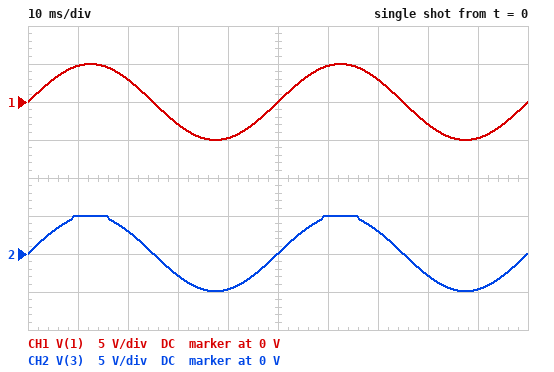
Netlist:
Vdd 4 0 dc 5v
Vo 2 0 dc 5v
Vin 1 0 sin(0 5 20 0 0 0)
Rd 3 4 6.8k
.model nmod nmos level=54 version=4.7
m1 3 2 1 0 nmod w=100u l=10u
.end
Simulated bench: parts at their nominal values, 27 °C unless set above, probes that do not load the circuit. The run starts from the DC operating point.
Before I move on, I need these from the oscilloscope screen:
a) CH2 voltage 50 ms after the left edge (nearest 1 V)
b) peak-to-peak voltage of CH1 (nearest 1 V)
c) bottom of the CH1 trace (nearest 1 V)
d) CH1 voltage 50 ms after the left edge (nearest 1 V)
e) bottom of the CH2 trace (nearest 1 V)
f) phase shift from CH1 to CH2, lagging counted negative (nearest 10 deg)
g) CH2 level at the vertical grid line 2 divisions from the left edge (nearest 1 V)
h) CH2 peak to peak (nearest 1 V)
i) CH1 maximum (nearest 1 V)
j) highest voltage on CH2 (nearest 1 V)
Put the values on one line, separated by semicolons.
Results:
0 V; 10 V; -5 V; 0 V; -5 V; 0 deg; 3 V; 10 V; 5 V; 5 V
